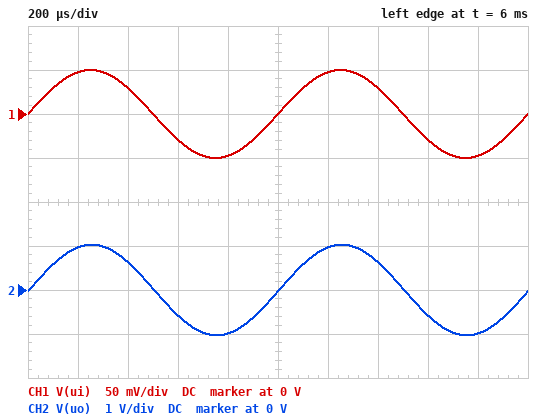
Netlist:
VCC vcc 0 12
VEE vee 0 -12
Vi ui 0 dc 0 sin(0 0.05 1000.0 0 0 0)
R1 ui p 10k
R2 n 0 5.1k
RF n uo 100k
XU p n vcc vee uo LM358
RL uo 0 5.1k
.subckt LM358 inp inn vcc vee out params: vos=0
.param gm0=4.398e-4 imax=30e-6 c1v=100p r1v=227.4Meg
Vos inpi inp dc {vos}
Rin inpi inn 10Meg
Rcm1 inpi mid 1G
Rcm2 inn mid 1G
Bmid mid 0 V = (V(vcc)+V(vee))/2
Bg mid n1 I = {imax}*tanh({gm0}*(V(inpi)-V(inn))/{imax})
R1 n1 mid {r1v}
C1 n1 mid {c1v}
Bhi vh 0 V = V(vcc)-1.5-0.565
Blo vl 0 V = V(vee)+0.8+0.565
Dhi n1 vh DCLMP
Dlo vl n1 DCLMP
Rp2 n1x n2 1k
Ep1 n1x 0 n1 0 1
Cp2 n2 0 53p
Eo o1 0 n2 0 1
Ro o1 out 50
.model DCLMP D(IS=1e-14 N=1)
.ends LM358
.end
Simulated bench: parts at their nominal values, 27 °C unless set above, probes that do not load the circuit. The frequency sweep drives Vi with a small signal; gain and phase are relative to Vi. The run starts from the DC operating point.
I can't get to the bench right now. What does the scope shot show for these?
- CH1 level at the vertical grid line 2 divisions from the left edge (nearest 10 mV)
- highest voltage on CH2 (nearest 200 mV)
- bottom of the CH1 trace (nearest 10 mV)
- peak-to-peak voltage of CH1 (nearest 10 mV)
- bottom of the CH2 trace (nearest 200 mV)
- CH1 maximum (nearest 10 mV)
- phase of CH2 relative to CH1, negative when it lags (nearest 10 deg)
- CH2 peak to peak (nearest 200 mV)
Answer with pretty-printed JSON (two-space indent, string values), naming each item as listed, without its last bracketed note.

{
  "CH1 level at the vertical grid line 2 divisions from the left edge": "30 mV",
  "highest voltage on CH2": "1.0 V",
  "bottom of the CH1 trace": "-50 mV",
  "peak-to-peak voltage of CH1": "100 mV",
  "bottom of the CH2 trace": "-1.0 V",
  "CH1 maximum": "50 mV",
  "phase of CH2 relative to CH1, negative when it lags": "0 deg",
  "CH2 peak to peak": "2.0 V"
}
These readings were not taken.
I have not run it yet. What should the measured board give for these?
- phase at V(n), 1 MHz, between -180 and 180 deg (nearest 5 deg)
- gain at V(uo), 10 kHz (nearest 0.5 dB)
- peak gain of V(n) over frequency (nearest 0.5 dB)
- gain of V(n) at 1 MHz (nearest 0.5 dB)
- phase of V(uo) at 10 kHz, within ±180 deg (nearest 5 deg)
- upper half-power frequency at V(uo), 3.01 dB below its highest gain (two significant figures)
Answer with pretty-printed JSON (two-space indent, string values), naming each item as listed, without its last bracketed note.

{
  "phase at V(n), 1 MHz, between -180 and 180 deg": "-105 deg",
  "gain at V(uo), 10 kHz": "26.0 dB",
  "peak gain of V(n) over frequency": "0 dB",
  "gain of V(n) at 1 MHz": "-30.0 dB",
  "phase of V(uo) at 10 kHz, within ±180 deg": "-15 deg",
  "upper half-power frequency at V(uo), 3.01 dB below its highest gain": "34 kHz"
}
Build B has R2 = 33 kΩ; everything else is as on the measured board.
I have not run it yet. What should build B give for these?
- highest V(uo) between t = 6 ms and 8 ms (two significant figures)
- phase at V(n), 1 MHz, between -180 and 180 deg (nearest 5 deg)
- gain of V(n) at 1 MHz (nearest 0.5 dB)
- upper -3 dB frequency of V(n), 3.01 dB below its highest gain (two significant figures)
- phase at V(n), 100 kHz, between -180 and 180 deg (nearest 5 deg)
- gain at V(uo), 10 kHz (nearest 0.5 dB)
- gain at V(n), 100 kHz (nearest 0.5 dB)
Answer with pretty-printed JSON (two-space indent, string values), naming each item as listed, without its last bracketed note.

{
  "highest V(uo) between t = 6 ms and 8 ms": "200 mV",
  "phase at V(n), 1 MHz, between -180 and 180 deg": "-100 deg",
  "gain of V(n) at 1 MHz": "-15.5 dB",
  "upper -3 dB frequency of V(n), 3.01 dB below its highest gain": "180 kHz",
  "phase at V(n), 100 kHz, between -180 and 180 deg": "-30 deg",
  "gain at V(uo), 10 kHz": "12.0 dB",
  "gain at V(n), 100 kHz": "-1.0 dB"
}
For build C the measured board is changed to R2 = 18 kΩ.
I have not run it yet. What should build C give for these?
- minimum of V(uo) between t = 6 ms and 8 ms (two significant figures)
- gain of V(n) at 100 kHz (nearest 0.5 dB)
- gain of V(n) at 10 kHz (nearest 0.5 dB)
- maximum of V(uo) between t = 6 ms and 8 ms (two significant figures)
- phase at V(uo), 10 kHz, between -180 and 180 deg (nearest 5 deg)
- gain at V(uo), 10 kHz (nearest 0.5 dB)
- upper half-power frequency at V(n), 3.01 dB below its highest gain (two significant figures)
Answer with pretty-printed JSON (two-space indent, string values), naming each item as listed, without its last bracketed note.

{
  "minimum of V(uo) between t = 6 ms and 8 ms": "-330 mV",
  "gain of V(n) at 100 kHz": "-2.5 dB",
  "gain of V(n) at 10 kHz": "0 dB",
  "maximum of V(uo) between t = 6 ms and 8 ms": "330 mV",
  "phase at V(uo), 10 kHz, between -180 and 180 deg": "-5 deg",
  "gain at V(uo), 10 kHz": "16.5 dB",
  "upper half-power frequency at V(n), 3.01 dB below its highest gain": "110 kHz"
}
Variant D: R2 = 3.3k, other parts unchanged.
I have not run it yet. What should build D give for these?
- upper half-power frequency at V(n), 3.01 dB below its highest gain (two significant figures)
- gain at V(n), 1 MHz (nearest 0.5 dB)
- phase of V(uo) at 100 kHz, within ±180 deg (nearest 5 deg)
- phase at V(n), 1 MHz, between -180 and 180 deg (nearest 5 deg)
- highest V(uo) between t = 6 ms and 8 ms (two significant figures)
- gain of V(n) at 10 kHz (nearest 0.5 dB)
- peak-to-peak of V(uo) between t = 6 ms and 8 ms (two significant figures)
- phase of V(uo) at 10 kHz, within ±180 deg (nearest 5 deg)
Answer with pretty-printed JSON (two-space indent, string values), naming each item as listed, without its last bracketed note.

{
  "upper half-power frequency at V(n), 3.01 dB below its highest gain": "22 kHz",
  "gain at V(n), 1 MHz": "-33.5 dB",
  "phase of V(uo) at 100 kHz, within ±180 deg": "-80 deg",
  "phase at V(n), 1 MHz, between -180 and 180 deg": "-105 deg",
  "highest V(uo) between t = 6 ms and 8 ms": "1.6 V",
  "gain of V(n) at 10 kHz": "-1.0 dB",
  "peak-to-peak of V(uo) between t = 6 ms and 8 ms": "3.1 V",
  "phase of V(uo) at 10 kHz, within ±180 deg": "-25 deg"
}
